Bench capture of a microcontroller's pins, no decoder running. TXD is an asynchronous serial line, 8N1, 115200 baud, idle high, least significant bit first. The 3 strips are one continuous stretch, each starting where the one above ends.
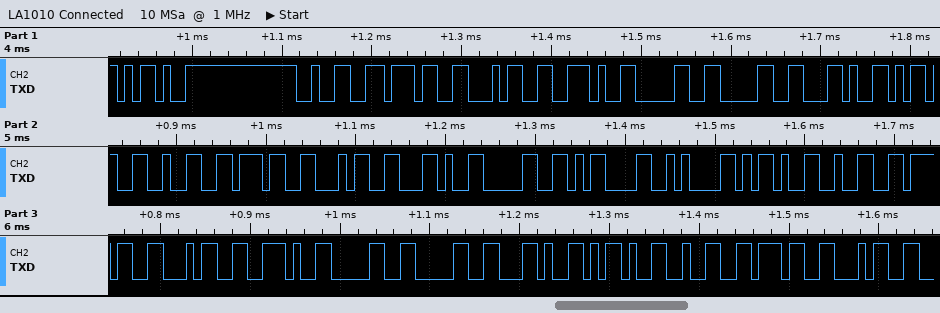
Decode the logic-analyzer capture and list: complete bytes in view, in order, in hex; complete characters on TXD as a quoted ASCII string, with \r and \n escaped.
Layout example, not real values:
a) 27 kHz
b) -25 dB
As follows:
a) 2D 32 37 34 2E 30 30 2C 2D 32 37 34 2C 30 0D 0A 2D 32 37 34 2E 30 30 2C 2D 32 37 34
b) "-274.00,-274,0\r\n-274.00,-274"
